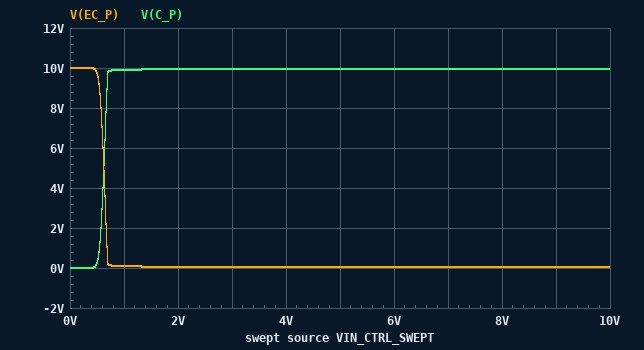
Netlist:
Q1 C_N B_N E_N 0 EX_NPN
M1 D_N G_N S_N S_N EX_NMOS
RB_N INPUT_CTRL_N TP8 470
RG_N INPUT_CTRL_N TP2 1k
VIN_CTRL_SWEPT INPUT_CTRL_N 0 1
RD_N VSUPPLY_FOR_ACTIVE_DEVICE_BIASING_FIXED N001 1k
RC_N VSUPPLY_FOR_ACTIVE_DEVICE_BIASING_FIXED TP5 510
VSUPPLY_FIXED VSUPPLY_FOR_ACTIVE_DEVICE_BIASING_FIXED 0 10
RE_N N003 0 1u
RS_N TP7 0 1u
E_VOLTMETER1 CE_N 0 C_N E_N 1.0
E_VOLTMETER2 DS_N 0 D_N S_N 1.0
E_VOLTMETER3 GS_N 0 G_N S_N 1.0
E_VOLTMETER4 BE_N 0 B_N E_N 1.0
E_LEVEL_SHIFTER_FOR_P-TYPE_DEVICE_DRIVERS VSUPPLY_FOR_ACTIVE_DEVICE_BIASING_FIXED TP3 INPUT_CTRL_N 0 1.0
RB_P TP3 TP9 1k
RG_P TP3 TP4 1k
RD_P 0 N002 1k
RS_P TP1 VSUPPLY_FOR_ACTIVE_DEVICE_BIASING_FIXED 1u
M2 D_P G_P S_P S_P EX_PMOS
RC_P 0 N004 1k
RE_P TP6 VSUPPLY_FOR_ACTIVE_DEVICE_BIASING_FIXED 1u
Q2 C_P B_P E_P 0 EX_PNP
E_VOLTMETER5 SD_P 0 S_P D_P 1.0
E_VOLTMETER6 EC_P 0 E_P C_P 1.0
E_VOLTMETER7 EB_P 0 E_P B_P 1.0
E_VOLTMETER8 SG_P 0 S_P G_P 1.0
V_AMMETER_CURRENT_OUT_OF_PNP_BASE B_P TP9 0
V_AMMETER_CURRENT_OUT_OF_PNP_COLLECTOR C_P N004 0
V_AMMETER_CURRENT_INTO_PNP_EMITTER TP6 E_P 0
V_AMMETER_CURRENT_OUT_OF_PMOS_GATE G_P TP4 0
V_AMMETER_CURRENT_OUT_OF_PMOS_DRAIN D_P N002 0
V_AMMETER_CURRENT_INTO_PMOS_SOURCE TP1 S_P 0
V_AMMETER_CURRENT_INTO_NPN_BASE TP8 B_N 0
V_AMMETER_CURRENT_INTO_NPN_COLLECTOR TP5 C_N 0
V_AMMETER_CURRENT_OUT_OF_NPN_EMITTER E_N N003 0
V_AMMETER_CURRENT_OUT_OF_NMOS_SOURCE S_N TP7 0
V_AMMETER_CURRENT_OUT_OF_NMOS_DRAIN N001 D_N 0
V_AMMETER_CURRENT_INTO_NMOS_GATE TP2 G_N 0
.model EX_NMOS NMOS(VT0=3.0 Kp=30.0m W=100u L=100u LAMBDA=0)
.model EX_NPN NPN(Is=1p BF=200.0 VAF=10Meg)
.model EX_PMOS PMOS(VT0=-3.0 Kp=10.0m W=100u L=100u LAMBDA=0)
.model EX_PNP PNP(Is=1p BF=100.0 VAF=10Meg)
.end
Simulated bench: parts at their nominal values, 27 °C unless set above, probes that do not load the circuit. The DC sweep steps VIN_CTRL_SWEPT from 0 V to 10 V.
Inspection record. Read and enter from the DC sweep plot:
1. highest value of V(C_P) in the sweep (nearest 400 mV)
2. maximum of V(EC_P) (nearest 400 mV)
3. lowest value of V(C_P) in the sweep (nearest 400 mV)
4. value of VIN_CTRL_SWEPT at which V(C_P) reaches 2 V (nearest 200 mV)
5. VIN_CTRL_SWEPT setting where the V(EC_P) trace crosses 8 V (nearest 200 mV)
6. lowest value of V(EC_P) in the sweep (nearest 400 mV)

10.0 V
10.0 V
0 V
600 mV
600 mV
0 V
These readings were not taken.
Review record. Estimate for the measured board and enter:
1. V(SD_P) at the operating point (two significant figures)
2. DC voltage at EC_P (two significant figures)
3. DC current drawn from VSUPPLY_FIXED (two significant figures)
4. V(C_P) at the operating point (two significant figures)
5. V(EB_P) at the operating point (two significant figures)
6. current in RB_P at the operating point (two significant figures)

10 V
92 mV
29 mA
9.9 V
600 mV
400 µA
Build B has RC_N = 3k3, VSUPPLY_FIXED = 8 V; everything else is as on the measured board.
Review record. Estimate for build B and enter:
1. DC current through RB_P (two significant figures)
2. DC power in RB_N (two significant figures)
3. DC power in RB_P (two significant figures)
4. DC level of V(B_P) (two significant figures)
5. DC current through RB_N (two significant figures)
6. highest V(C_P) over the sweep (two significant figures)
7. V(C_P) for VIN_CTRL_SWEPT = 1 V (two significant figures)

410 µA
390 µW
170 µW
7.4 V
910 µA
8.0 V
7.9 V
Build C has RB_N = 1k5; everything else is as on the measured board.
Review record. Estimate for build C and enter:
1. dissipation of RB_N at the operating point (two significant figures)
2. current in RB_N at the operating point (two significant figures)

100 µW
260 µA
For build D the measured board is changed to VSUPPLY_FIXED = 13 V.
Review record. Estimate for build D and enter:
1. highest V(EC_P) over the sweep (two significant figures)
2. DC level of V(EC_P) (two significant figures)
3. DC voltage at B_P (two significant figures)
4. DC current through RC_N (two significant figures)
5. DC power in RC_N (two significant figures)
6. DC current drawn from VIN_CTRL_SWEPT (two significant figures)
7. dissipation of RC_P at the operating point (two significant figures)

13 V
100 mV
12 V
25 mA
330 mW
810 µA
170 mW
